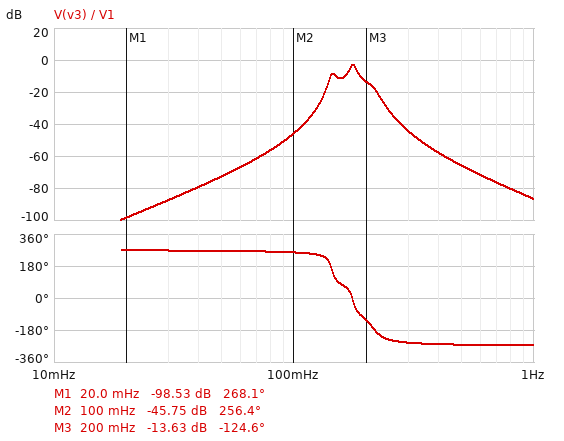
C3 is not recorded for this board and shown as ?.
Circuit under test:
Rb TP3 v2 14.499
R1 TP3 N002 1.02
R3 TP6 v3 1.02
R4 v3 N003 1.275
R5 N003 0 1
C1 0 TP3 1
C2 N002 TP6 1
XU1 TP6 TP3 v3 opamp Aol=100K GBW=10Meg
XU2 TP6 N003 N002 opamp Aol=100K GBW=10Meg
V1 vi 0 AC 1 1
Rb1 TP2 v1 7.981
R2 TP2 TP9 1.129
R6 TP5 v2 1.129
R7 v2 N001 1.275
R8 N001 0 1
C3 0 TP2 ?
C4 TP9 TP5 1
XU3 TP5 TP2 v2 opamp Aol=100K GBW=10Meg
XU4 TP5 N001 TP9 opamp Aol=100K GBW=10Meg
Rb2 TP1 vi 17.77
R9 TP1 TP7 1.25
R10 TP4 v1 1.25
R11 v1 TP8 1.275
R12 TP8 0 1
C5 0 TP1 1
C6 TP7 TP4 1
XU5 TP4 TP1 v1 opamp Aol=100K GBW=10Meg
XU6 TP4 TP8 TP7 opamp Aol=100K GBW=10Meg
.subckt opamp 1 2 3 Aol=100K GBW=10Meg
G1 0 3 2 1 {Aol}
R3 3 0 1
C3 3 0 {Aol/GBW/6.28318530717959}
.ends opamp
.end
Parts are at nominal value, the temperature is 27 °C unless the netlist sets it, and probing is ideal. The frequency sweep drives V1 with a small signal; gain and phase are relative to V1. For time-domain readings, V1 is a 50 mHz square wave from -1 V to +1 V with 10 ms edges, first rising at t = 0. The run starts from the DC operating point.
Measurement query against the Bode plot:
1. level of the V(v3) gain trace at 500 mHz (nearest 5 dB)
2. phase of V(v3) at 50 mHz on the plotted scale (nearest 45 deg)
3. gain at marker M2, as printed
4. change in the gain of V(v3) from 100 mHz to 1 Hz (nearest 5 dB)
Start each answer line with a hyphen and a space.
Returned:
- -65 dB
- 270 deg
- -45.75 dB
- -40 dB
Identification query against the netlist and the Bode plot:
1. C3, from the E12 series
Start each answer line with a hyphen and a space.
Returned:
- 560 mF
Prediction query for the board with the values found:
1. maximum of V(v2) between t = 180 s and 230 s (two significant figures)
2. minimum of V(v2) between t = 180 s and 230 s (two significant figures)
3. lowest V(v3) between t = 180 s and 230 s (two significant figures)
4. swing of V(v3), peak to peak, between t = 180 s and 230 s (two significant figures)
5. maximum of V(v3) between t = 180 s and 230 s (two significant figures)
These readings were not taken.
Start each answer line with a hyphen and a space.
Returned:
- 330 mV
- -330 mV
- -130 mV
- 270 mV
- 130 mV
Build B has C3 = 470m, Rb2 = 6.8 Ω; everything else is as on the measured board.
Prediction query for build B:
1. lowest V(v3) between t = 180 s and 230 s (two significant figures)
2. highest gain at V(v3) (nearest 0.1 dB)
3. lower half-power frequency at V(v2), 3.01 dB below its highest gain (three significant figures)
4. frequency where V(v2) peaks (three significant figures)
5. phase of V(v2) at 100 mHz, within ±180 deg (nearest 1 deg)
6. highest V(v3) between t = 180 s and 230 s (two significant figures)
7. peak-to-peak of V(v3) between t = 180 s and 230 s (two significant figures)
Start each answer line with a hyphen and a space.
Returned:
- -190 mV
- 2.6 dB
- 136 mHz
- 146 mHz
- 162 deg
- 190 mV
- 390 mV
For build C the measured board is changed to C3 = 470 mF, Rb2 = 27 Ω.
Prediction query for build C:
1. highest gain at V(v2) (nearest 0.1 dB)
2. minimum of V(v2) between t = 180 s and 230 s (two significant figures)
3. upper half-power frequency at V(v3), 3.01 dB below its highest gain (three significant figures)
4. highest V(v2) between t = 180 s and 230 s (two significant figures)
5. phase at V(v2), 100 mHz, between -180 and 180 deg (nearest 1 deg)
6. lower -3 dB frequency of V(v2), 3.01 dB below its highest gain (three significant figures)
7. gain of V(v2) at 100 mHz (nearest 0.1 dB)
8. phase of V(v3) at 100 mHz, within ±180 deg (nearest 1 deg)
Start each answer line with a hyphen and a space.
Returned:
- -0.6 dB
- -230 mV
- 181 mHz
- 230 mV
- 171 deg
- 141 mHz
- -31.2 dB
- -102 deg
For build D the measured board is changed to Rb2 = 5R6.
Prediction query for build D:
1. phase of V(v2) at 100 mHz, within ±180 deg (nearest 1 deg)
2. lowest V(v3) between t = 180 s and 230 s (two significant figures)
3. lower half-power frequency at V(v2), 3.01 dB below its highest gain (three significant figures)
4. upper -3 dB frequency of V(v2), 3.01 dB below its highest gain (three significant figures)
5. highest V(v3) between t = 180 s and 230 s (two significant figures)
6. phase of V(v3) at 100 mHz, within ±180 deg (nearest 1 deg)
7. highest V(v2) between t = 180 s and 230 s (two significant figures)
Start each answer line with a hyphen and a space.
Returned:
- 159 deg
- -220 mV
- 138 mHz
- 225 mHz
- 220 mV
- -114 deg
- 550 mV
